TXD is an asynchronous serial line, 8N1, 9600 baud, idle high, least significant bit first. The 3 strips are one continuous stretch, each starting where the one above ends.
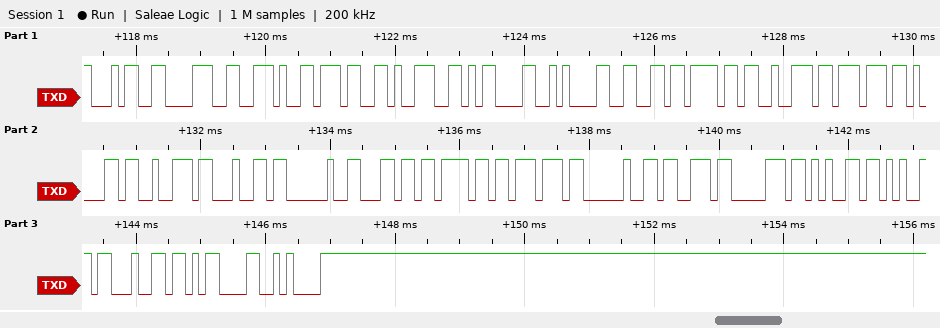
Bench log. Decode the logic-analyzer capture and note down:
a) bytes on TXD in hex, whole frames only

34 38 2E 37 39 0D 0A 66 6F 72 77 61 72 64 20 6C 6F 77 20 73 70 65 65 64 0D 0A
